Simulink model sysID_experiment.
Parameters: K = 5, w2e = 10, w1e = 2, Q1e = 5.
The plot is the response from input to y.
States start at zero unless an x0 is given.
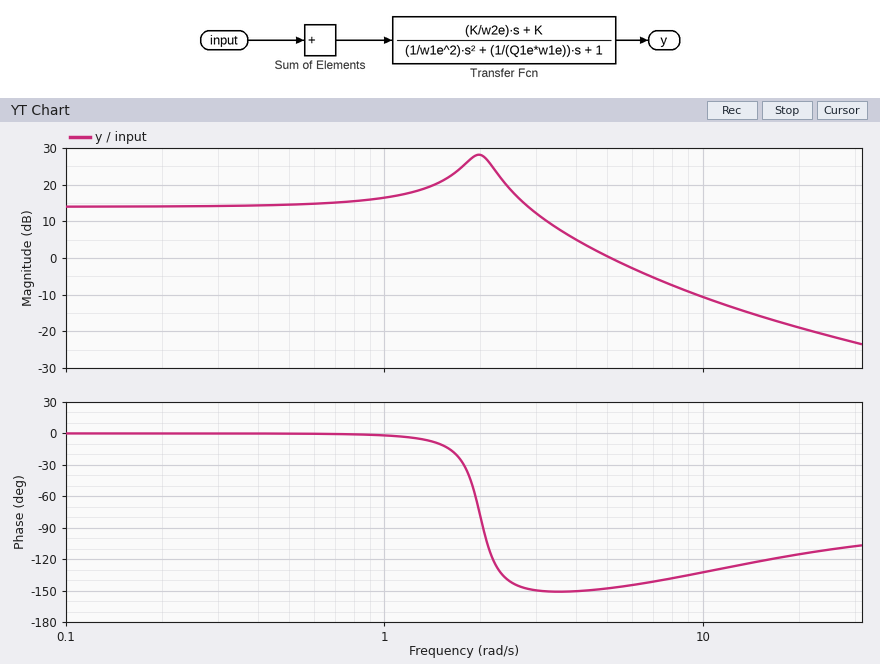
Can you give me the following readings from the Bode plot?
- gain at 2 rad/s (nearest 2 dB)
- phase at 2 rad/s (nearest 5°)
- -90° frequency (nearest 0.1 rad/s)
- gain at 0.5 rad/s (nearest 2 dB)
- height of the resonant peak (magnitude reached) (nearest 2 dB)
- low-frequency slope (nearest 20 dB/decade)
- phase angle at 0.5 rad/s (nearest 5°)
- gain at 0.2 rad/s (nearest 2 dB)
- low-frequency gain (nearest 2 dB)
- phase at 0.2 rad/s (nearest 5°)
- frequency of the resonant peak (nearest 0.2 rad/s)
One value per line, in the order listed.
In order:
28 dB
-80°
2.0 rad/s
14 dB
28 dB
0 dB/decade
0°
14 dB
14 dB
0°
2.0 rad/s
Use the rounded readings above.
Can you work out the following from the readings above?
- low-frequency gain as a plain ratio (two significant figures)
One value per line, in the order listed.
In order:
5.0
